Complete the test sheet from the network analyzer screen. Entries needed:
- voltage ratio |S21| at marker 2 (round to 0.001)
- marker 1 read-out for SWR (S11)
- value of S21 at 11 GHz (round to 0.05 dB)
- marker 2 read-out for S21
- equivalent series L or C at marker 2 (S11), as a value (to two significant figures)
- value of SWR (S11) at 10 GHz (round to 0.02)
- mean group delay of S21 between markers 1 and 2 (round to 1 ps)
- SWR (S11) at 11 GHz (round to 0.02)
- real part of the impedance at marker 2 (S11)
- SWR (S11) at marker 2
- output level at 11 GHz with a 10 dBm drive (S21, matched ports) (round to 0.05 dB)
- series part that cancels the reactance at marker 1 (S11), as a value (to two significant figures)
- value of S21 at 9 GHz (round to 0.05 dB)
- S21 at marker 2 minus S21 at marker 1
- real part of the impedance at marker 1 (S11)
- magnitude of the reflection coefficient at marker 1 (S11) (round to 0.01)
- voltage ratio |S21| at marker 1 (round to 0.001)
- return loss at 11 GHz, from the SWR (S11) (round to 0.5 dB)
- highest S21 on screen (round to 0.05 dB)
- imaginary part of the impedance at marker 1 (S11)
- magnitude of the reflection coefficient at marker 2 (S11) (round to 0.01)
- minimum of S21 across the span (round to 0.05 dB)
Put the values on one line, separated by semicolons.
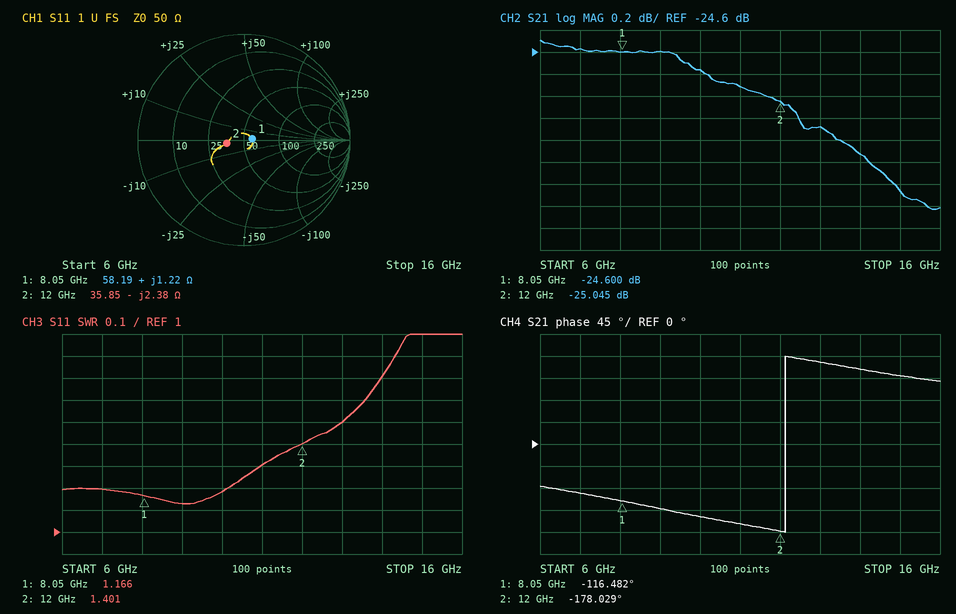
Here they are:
0.056; 1.166; -24.90 dB; -25.045 dB; 5.6 pF; 1.18; 43 ps; 1.30; 35.85 Ω; 1.401; -14.90 dBm; 16 pF; -24.60 dB; -0.445 dB; 58.19 Ω; 0.08; 0.059; 17.5 dB; -24.50 dB; +1.22 Ω; 0.17; -26.05 dB
